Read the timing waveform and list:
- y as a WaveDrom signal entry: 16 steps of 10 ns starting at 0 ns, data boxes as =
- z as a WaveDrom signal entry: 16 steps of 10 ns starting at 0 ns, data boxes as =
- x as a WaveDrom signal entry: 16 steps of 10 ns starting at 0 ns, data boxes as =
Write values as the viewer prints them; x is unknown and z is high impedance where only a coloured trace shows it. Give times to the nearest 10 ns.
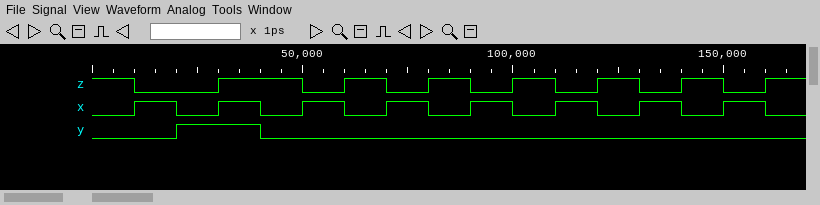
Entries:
{name: 'y', wave: '0.1.0...........'}
{name: 'z', wave: '10.1.01010101010'}
{name: 'x', wave: '0101010101010101'}
